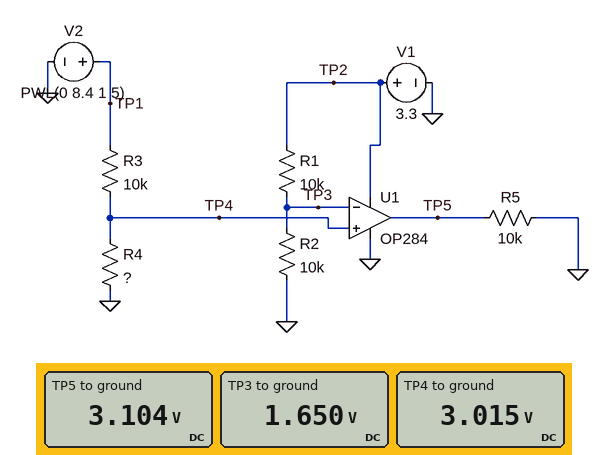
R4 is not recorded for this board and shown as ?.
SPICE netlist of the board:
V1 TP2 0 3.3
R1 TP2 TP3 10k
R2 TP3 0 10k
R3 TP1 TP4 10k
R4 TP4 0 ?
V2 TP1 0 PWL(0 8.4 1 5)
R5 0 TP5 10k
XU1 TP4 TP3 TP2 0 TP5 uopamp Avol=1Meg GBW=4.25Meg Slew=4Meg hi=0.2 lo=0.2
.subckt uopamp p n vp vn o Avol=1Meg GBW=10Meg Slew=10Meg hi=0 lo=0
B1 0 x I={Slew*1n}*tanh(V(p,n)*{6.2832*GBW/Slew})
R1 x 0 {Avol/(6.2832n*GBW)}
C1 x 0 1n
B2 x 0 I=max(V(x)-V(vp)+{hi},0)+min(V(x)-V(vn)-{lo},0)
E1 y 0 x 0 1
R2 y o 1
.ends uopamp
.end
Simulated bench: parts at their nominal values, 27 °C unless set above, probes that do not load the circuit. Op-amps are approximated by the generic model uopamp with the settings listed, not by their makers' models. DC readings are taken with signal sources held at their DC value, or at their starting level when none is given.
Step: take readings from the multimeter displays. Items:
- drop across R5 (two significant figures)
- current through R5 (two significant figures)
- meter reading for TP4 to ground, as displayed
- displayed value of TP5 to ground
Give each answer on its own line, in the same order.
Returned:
3.1 V
310 µA
3.015 V
3.104 V
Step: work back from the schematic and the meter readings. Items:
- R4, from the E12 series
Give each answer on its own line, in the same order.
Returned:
5.6 kΩ
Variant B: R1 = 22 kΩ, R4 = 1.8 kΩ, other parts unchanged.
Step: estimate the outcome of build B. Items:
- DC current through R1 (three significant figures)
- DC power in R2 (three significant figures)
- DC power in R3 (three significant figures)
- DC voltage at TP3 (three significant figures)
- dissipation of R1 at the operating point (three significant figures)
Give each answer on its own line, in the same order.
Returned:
103 µA
106 µW
5.07 mW
1.03 V
234 µW
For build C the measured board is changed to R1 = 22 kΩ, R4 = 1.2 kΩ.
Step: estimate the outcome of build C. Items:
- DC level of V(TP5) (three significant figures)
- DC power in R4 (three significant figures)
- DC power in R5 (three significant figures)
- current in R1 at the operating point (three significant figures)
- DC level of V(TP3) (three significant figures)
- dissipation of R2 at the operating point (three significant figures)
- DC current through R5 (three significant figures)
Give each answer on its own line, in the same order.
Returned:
197 mV
675 µW
3.89 µW
103 µA
1.03 V
106 µW
19.7 µA
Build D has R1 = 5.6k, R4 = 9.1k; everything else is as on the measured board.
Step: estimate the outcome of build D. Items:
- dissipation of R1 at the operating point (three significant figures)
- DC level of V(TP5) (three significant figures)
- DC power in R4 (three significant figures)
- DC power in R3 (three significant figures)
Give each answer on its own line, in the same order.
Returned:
251 µW
3.10 V
1.76 mW
1.93 mW
